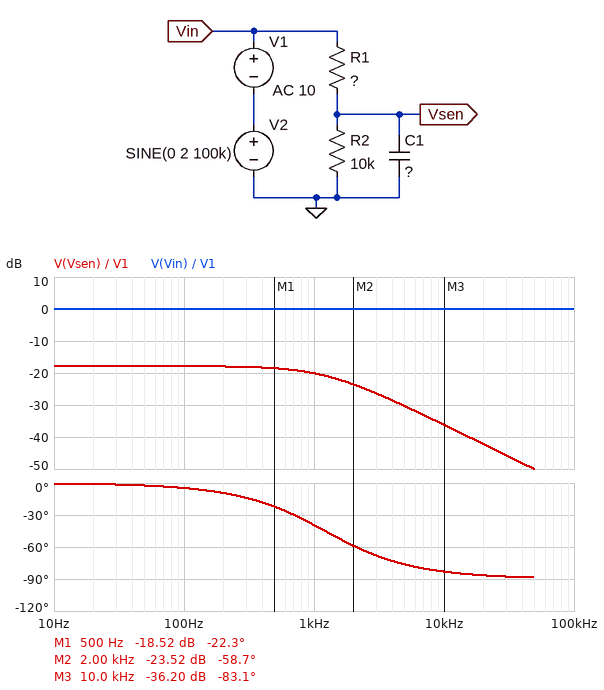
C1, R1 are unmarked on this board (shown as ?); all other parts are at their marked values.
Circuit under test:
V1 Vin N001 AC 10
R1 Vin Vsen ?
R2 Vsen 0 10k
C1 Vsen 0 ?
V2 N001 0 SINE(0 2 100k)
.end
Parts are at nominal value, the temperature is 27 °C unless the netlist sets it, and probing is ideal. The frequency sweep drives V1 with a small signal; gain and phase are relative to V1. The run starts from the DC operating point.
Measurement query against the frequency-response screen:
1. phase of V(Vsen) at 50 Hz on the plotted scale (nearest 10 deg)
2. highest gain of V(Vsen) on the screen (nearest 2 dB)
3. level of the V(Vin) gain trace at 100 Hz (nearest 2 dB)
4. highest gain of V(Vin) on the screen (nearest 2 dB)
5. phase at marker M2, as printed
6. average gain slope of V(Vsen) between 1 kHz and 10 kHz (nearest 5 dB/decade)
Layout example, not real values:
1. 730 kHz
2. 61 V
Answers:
1. 0 deg
2. -18 dB
3. 0 dB
4. 0 dB
5. -58.7 deg
6. -15 dB/decade
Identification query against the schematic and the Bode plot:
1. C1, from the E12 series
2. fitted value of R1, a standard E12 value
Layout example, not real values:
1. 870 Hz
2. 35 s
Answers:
1. 15 nF
2. 68 kΩ
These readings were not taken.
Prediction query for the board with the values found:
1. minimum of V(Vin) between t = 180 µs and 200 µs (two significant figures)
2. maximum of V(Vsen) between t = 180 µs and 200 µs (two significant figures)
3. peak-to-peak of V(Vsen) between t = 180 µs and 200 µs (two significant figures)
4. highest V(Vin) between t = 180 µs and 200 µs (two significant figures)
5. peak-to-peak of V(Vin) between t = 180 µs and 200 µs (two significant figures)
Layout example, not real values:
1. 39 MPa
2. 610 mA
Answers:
1. -2.0 V
2. 3.9 mV
3. 6.3 mV
4. 2.0 V
5. 4.0 V
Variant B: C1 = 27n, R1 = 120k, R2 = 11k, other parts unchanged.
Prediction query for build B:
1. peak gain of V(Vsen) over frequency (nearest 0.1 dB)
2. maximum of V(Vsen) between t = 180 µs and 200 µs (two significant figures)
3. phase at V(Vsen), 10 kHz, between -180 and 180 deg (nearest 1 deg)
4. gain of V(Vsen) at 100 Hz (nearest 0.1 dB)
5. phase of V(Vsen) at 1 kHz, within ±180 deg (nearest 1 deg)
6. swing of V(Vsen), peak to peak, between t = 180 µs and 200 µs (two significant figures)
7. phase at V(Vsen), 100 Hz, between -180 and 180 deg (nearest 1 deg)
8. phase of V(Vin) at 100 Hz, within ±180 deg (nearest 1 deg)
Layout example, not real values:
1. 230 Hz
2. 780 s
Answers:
1. -21.5 dB
2. 1.5 mV
3. -87 deg
4. -21.6 dB
5. -60 deg
6. 2.0 mV
7. -10 deg
8. 0 deg
